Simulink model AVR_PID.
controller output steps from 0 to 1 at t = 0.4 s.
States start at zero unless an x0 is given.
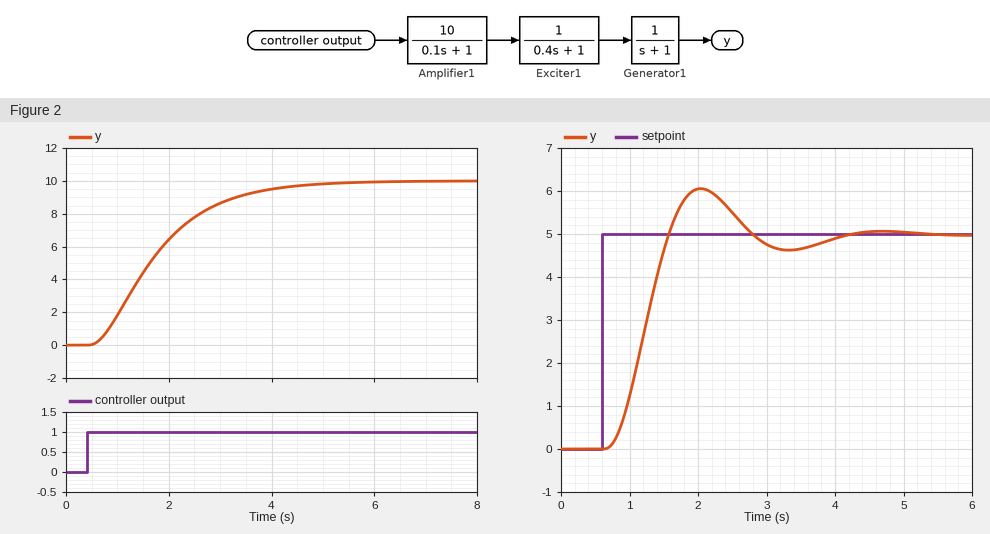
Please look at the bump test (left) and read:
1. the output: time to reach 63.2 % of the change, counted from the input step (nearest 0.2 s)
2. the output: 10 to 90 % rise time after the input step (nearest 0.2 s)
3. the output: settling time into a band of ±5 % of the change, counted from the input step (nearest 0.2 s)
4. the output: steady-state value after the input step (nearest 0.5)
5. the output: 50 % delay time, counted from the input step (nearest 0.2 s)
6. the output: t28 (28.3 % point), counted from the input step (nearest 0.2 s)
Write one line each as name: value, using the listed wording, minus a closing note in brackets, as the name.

the output: time to reach 63.2 % of the change, counted from the input step: 1.6 s
the output: 10 to 90 % rise time after the input step: 2.4 s
the output: settling time into a band of ±5 % of the change, counted from the input step: 3.6 s
the output: steady-state value after the input step: 10.0
the output: 50 % delay time, counted from the input step: 1.2 s
the output: t28 (28.3 % point), counted from the input step: 0.8 s
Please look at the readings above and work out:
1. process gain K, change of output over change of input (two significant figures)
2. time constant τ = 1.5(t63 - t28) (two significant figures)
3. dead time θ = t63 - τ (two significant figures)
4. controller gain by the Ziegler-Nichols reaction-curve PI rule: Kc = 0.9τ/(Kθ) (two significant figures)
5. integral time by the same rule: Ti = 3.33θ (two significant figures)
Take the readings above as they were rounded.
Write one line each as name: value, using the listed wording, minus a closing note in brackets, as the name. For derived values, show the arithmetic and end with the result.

process gain K, change of output over change of input: (10 - 0) / 1 = 10
time constant τ = 1.5(t63 - t28): 1.5 × (1.6 - 0.8) = 1.2 s
dead time θ = t63 - τ: 1.6 - 1.2 = 0.40 s
controller gain by the Ziegler-Nichols reaction-curve PI rule: Kc = 0.9τ/(Kθ): 0.9 × 1.2 / (10 × 0.4) = 0.27
integral time by the same rule: Ti = 3.33θ: 3.33 × 0.4 = 1.3 s
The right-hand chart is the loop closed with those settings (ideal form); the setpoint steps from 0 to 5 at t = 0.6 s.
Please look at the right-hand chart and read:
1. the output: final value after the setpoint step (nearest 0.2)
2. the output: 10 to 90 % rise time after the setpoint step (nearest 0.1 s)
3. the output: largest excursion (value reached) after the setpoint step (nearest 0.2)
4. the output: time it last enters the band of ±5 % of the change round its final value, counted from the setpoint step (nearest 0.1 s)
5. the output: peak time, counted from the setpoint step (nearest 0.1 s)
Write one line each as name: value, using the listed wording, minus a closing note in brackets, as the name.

the output: final value after the setpoint step: 5.0
the output: 10 to 90 % rise time after the setpoint step: 0.6 s
the output: largest excursion (value reached) after the setpoint step: 6.0
the output: time it last enters the band of ±5 % of the change round its final value, counted from the setpoint step: 3.1 s
the output: peak time, counted from the setpoint step: 1.4 s
